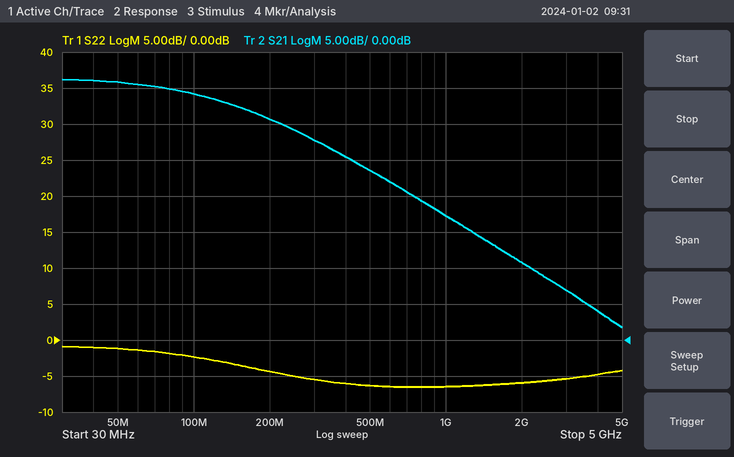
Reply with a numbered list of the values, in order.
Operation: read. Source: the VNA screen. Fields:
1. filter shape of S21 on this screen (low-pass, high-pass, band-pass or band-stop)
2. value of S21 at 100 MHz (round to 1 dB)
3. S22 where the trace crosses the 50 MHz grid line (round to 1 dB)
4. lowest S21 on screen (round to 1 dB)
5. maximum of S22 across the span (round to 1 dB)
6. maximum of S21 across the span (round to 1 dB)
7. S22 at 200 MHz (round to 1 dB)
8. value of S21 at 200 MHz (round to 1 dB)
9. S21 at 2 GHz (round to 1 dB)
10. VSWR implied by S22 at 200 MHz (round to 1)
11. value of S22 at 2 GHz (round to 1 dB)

1. low-pass
2. 34 dB
3. -1 dB
4. 2 dB
5. -1 dB
6. 36 dB
7. -4 dB
8. 31 dB
9. 11 dB
10. 4
11. -6 dB
